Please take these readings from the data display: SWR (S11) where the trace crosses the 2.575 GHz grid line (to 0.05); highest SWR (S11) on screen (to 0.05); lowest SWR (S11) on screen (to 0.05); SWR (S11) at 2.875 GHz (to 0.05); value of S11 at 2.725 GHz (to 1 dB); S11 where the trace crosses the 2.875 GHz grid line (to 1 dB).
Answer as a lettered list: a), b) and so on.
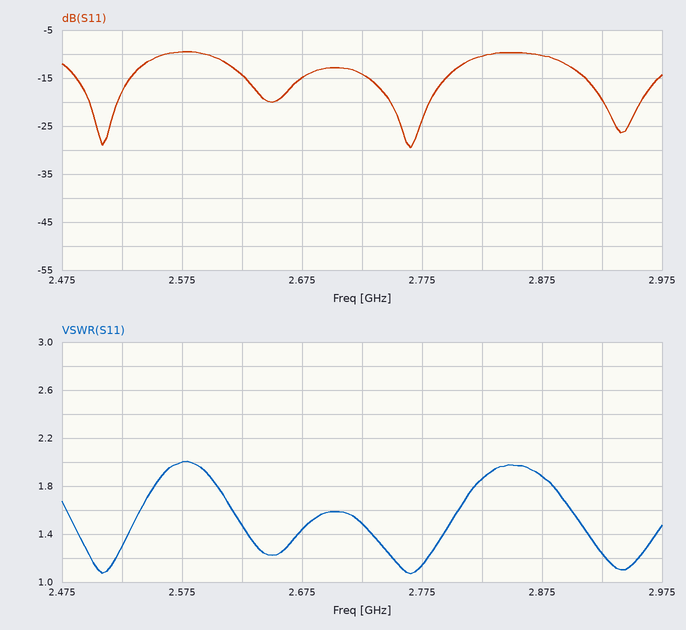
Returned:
a) 2.00
b) 2.00
c) 1.05
d) 1.90
e) -14 dB
f) -10 dB
